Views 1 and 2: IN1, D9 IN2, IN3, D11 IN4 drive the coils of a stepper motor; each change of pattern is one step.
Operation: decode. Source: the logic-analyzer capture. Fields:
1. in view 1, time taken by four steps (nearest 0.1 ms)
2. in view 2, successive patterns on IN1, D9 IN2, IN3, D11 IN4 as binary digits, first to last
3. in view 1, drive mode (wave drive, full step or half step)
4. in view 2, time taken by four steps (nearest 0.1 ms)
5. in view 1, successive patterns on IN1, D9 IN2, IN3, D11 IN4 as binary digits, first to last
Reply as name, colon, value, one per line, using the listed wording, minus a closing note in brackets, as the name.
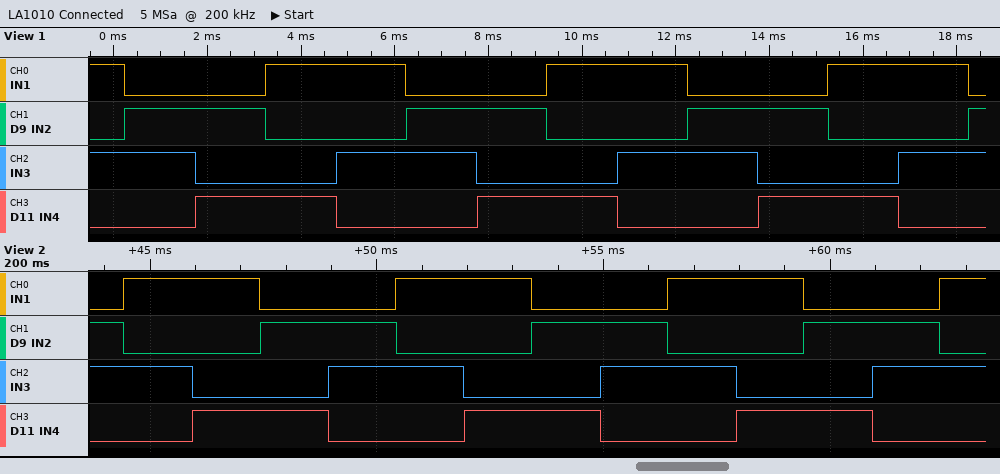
in view 1, time taken by four steps: 6.0 ms
in view 2, successive patterns on IN1, D9 IN2, IN3, D11 IN4 as binary digits, first to last: 0110 1010 1001 0101 0110 1010 1001 0101 0110 1010 1001 0101 0110 1010
in view 1, drive mode: full step
in view 2, time taken by four steps: 6.0 ms
in view 1, successive patterns on IN1, D9 IN2, IN3, D11 IN4 as binary digits, first to last: 1010 0110 0101 1001 1010 0110 0101 1001 1010 0110 0101 1001 1010 0110
